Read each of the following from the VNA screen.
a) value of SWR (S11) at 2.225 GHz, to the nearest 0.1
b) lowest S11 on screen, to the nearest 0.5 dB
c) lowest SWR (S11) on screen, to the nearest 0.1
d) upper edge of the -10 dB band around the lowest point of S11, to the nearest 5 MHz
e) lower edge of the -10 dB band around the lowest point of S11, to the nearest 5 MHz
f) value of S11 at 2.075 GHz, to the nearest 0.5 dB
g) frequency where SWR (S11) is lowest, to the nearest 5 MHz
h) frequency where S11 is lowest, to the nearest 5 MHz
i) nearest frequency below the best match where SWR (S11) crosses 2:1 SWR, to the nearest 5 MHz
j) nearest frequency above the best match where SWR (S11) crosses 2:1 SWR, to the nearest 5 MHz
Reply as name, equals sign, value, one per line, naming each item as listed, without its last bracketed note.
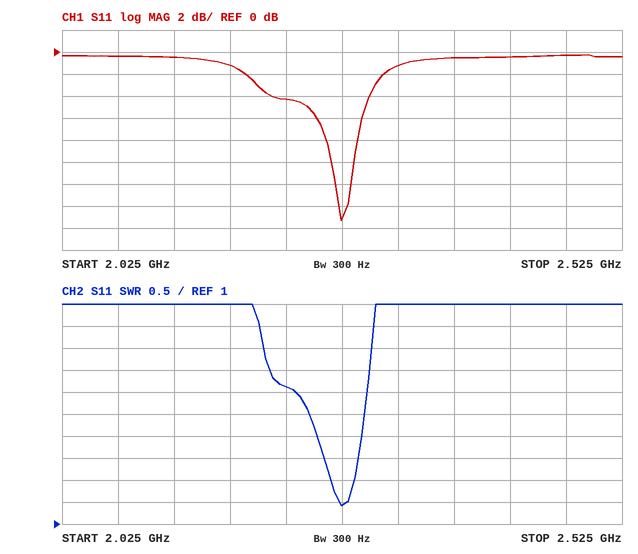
value of SWR (S11) at 2.225 GHz, to the nearest 0.1 = 4.1
lowest S11 on screen, to the nearest 0.5 dB = -15.5 dB
lowest SWR (S11) on screen, to the nearest 0.1 = 1.4
upper edge of the -10 dB band around the lowest point of S11, to the nearest 5 MHz = 2.285 GHz
lower edge of the -10 dB band around the lowest point of S11, to the nearest 5 MHz = 2.265 GHz
value of S11 at 2.075 GHz, to the nearest 0.5 dB = -0.5 dB
frequency where SWR (S11) is lowest, to the nearest 5 MHz = 2.275 GHz
frequency where S11 is lowest, to the nearest 5 MHz = 2.275 GHz
nearest frequency below the best match where SWR (S11) crosses 2:1 SWR, to the nearest 5 MHz = 2.265 GHz
nearest frequency above the best match where SWR (S11) crosses 2:1 SWR, to the nearest 5 MHz = 2.285 GHz
